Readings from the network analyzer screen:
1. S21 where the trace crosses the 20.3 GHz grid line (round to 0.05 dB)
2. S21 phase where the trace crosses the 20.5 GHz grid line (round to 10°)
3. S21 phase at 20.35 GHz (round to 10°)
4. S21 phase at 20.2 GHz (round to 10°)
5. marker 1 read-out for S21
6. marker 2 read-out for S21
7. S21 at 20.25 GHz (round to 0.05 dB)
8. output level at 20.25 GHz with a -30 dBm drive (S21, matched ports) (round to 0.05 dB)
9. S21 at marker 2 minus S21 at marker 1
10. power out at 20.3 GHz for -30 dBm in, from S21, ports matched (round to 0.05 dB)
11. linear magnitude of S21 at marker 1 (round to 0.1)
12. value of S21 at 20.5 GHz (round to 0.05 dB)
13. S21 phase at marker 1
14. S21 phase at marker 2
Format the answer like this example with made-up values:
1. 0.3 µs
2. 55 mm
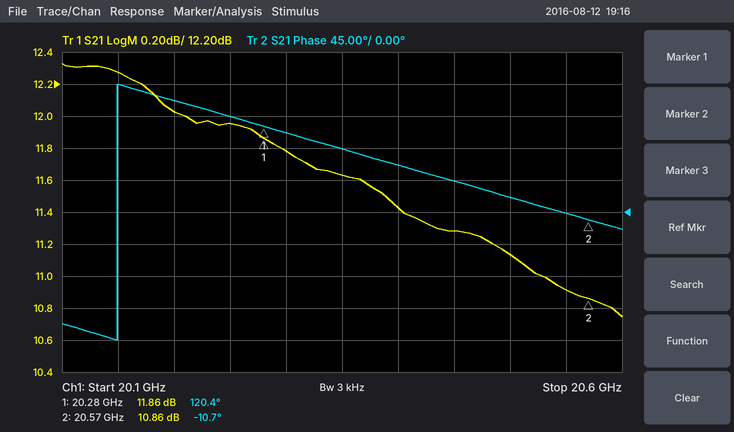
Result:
1. 11.80 dB
2. 20°
3. 90°
4. 160°
5. 11.86 dB
6. 10.86 dB
7. 11.95 dB
8. -18.05 dBm
9. -1.00 dB
10. -18.20 dBm
11. 3.9
12. 11.15 dB
13. 120.4°
14. -10.7°
